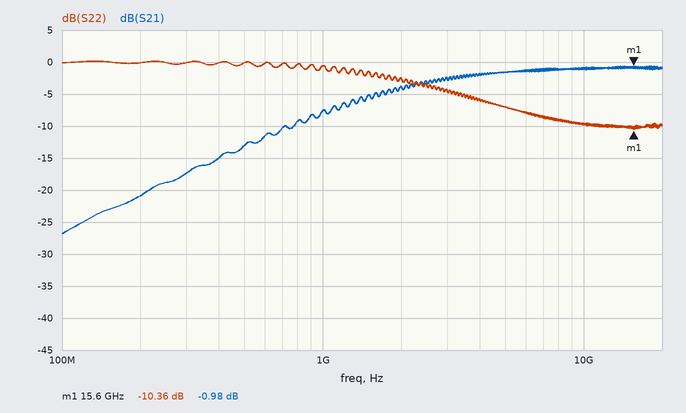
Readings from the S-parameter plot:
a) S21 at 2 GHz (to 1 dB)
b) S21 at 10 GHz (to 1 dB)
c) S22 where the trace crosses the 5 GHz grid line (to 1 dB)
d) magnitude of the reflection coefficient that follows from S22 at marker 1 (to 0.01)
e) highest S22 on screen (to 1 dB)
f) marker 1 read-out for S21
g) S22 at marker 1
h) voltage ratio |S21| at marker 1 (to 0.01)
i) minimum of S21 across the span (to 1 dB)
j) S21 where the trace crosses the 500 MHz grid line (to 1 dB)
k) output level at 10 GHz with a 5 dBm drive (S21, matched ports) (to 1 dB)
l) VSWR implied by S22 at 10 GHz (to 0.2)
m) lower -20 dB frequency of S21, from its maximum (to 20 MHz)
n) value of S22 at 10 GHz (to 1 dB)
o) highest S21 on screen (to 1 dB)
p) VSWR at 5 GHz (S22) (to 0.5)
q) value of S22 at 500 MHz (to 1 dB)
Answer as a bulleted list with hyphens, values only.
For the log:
- -4 dB
- -1 dB
- -7 dB
- 0.30
- 0 dB
- -0.98 dB
- -10.36 dB
- 0.89
- -27 dB
- -13 dB
- 4 dBm
- 2.0
- 200 MHz
- -10 dB
- -1 dB
- 2.5
- 0 dB
